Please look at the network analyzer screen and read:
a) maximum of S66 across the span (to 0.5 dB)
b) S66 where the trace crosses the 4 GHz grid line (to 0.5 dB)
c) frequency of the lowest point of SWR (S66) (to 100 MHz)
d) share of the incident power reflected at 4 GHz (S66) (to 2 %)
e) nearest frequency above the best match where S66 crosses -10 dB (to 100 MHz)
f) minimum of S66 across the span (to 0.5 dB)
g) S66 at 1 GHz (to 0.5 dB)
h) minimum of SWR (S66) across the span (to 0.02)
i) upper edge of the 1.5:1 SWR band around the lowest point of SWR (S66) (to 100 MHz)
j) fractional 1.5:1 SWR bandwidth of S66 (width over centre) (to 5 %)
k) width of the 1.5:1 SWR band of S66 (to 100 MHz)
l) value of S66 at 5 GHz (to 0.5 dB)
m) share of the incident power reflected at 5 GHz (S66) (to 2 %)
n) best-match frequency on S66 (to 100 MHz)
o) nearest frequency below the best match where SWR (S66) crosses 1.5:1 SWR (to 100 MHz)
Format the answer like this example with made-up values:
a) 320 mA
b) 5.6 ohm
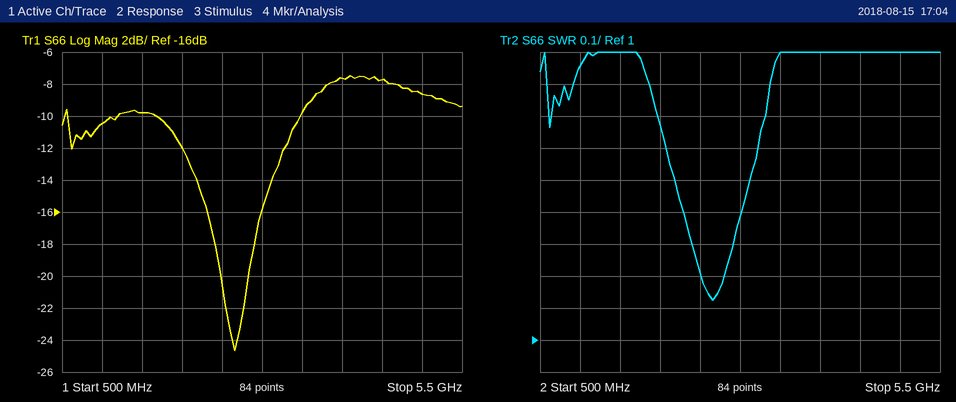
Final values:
a) -7.5 dB
b) -7.5 dB
c) 2.7 GHz
d) 18 %
e) 3.5 GHz
f) -24.5 dB
g) -10.5 dB
h) 1.12
i) 3.1 GHz
j) 35 %
k) 900 MHz
l) -8.5 dB
m) 14 %
n) 2.7 GHz
o) 2.2 GHz
